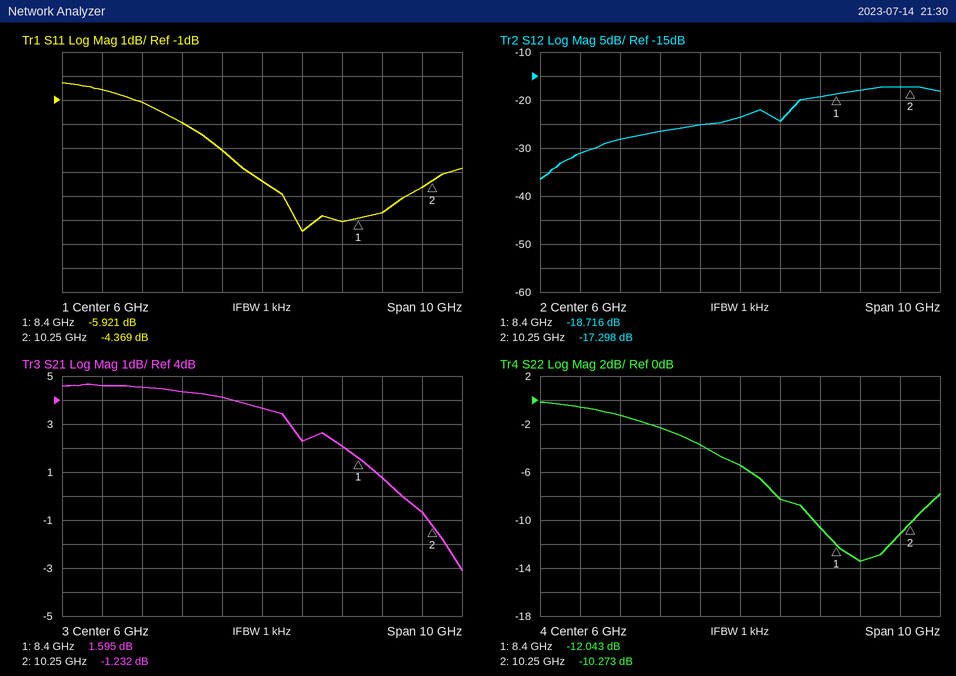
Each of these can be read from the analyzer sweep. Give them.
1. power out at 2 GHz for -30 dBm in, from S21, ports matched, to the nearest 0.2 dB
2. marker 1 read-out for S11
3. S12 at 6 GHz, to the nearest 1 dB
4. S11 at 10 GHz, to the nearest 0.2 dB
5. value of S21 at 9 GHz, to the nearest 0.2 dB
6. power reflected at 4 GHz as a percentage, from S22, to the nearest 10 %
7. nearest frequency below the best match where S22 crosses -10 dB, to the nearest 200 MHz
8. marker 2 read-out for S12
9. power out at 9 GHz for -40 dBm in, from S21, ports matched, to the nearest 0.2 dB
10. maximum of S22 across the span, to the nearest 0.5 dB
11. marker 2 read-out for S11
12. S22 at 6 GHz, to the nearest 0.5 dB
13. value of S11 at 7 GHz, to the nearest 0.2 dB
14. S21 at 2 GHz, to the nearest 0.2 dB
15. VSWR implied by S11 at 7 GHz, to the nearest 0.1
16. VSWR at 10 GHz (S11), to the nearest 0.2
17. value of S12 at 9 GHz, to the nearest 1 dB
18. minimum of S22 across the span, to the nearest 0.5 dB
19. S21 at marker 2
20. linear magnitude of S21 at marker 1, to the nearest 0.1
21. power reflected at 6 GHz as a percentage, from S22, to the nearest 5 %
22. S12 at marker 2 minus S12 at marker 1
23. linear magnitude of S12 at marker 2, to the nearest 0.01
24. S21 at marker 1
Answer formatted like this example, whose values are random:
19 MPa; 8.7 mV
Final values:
-25.4 dBm; -5.921 dB; -24 dB; -4.6 dB; 0.8 dB; 60 %; 7.8 GHz; -17.298 dB; -39.2 dBm; 0.0 dB; -4.369 dB; -5.5 dB; -6.4 dB; 4.6 dB; 2.8; 3.8; -18 dB; -13.5 dB; -1.232 dB; 1.2; 30 %; 1.418 dB; 0.14; 1.595 dB
